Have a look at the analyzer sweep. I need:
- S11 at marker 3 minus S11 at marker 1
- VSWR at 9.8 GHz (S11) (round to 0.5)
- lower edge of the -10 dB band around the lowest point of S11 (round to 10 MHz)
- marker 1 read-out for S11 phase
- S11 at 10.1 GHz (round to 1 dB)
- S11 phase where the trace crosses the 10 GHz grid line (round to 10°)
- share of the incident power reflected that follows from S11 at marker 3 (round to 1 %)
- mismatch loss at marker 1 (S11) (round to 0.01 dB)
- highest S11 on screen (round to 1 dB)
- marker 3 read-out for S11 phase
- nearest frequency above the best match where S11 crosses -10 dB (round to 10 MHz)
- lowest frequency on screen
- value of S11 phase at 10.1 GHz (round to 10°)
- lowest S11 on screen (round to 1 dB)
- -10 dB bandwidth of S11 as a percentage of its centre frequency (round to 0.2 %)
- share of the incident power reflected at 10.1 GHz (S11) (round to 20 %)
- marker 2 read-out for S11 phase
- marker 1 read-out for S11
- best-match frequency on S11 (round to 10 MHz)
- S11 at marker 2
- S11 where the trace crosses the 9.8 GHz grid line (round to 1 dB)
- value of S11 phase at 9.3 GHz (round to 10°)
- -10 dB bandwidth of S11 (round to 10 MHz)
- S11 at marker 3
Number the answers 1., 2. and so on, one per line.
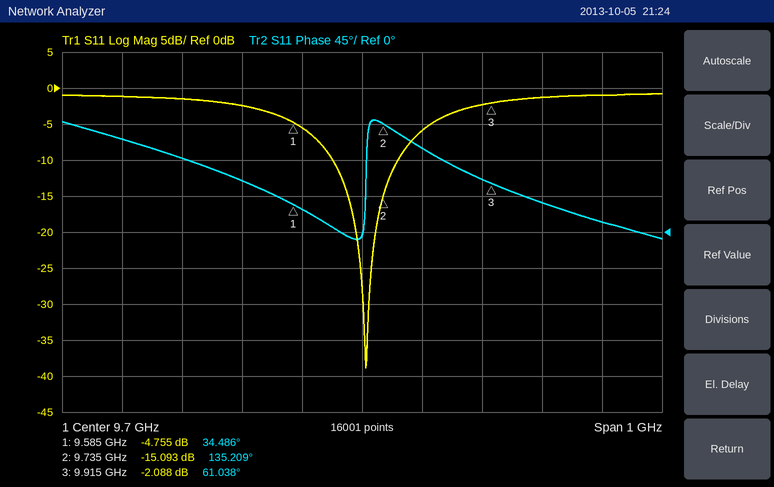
1. 2.667 dB
2. 3.0
3. 9.65 GHz
4. 34.486°
5. -1 dB
6. 40°
7. 62 %
8. 1.77 dB
9. -1 dB
10. 61.038°
11. 9.76 GHz
12. 9.2 GHz
13. 10°
14. -39 dB
15. 1.2 %
16. 80 %
17. 135.209°
18. -4.755 dB
19. 9.71 GHz
20. -15.093 dB
21. -6 dB
22. 120°
23. 110 MHz
24. -2.088 dB
